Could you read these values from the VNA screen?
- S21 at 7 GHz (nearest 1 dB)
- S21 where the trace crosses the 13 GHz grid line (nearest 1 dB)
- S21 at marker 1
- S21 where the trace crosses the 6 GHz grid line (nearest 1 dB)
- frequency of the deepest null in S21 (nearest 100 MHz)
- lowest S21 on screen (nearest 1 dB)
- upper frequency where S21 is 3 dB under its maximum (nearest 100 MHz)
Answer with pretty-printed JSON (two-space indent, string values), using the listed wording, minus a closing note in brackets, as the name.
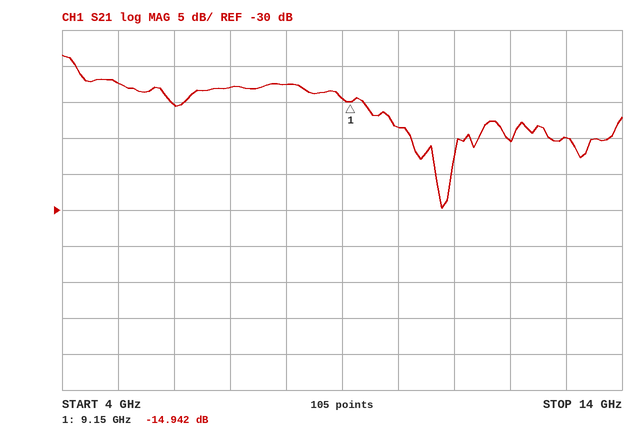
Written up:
{
  "S21 at 7 GHz": "-13 dB",
  "S21 where the trace crosses the 13 GHz grid line": "-20 dB",
  "S21 at marker 1": "-14.942 dB",
  "S21 where the trace crosses the 6 GHz grid line": "-15 dB",
  "frequency of the deepest null in S21": "10.8 GHz",
  "lowest S21 on screen": "-30 dB",
  "upper frequency where S21 is 3 dB under its maximum": "4.4 GHz"
}
